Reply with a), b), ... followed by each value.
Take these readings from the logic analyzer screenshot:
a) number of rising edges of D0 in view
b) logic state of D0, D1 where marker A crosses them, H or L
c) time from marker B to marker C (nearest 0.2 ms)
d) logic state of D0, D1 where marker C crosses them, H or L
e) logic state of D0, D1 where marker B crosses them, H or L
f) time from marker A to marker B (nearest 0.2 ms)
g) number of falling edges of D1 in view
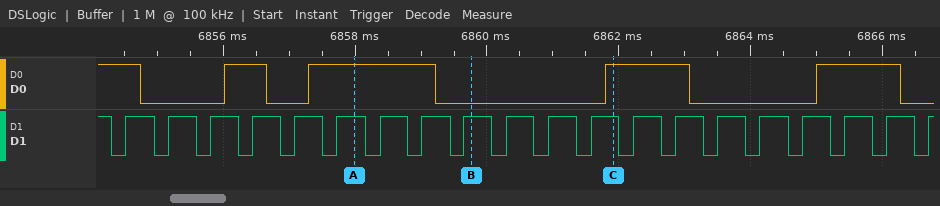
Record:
a) 4
b) D0=H, D1=H
c) 2.2 ms
d) D0=H, D1=H
e) D0=L, D1=H
f) 1.8 ms
g) 20
